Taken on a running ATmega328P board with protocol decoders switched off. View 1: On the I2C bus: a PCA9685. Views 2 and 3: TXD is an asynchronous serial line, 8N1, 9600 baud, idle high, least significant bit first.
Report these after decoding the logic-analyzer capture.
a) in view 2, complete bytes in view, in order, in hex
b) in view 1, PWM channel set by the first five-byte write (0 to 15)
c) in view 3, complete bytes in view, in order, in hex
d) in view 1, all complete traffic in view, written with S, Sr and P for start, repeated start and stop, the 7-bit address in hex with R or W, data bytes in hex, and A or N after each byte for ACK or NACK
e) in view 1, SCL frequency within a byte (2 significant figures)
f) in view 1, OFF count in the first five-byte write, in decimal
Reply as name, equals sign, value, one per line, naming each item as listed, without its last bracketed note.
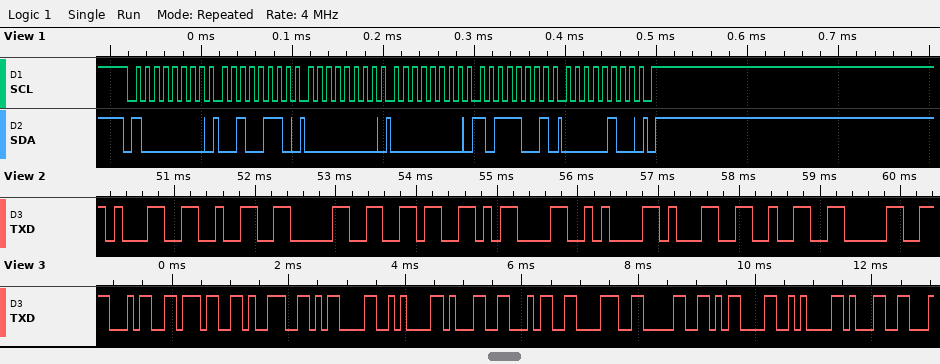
in view 2, complete bytes in view, in order, in hex = 31 32 30 36 0D 0A 31 32 30
in view 1, PWM channel set by the first five-byte write = 8
in view 3, complete bytes in view, in order, in hex = 0x34 0x37 0x39 0x0D 0x0A 0x31 0x34 0x38 0x30 0x0D 0x0A 0x31
in view 1, all complete traffic in view, written with S, Sr and P for start, repeated start and stop, the 7-bit address in hex with R or W, data bytes in hex, and A or N after each byte for ACK or NACK = S 40W A 26 A 00 A 00 A B9 A 04 A P
in view 1, SCL frequency within a byte = 100 kHz
in view 1, OFF count in the first five-byte write, in decimal = 1209
